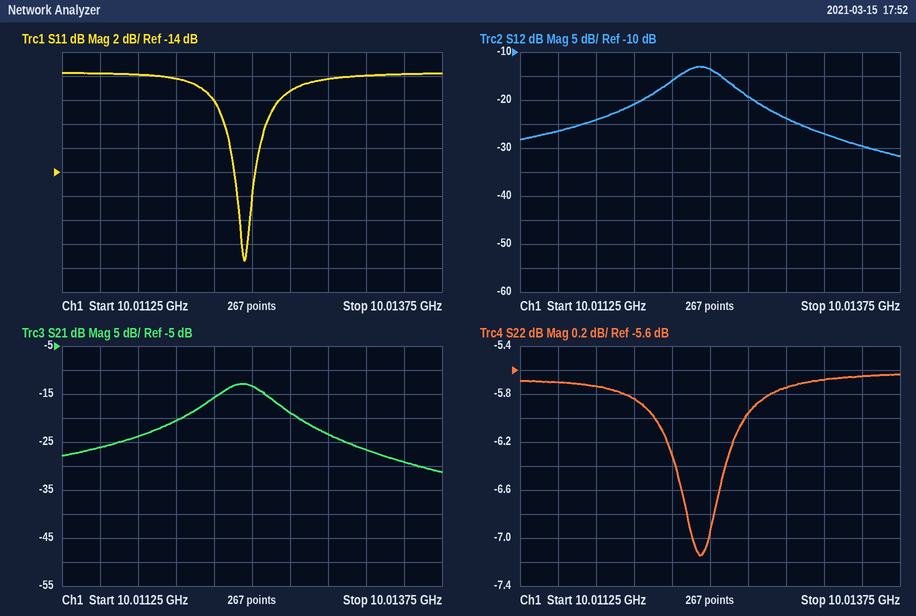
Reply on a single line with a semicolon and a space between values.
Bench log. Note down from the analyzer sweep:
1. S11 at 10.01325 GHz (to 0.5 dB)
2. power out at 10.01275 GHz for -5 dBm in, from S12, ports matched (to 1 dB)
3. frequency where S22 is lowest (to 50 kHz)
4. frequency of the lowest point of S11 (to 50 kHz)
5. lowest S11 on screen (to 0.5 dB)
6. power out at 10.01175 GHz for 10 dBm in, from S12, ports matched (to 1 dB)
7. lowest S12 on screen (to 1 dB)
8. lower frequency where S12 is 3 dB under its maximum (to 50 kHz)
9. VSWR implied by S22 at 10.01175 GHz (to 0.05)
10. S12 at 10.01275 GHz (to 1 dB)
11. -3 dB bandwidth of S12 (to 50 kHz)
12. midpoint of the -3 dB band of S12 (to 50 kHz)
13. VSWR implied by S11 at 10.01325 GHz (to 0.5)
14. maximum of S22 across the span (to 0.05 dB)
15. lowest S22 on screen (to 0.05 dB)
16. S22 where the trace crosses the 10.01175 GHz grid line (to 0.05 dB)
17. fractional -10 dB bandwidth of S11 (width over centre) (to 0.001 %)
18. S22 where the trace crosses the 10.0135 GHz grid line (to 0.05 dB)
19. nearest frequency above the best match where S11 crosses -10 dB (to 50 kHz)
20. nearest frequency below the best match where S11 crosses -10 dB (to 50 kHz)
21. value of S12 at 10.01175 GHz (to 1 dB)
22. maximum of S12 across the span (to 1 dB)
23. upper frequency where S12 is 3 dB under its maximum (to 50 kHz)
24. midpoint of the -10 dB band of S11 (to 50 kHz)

-6.0 dB; -24 dBm; 10.01245 GHz; 10.01245 GHz; -21.5 dB; -14 dBm; -32 dB; 10.01225 GHz; 3.15; -19 dB; 350 kHz; 10.01245 GHz; 3.0; -5.65 dB; -7.15 dB; -5.75 dB; 0.003 %; -5.65 dB; 10.01260 GHz; 10.01230 GHz; -24 dB; -13 dB; 10.01260 GHz; 10.01245 GHz
